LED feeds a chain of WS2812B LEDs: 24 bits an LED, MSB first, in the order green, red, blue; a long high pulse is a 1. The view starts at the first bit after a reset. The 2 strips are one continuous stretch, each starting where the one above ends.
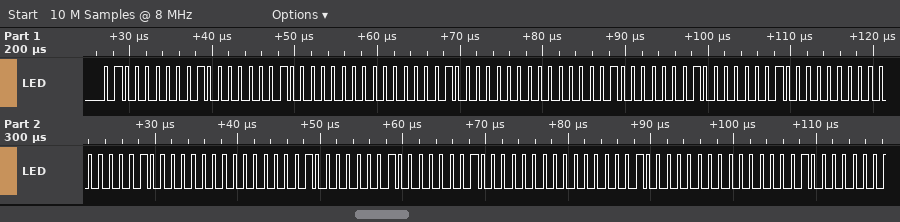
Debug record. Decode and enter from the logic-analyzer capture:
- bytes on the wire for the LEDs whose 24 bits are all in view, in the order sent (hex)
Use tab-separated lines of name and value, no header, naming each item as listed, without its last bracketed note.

bytes on the wire for the LEDs whose 24 bits are all in view, in the order sent	40 40 40 00 40 00 40 40 40 00 40 00 40 40 40 00 40 00
